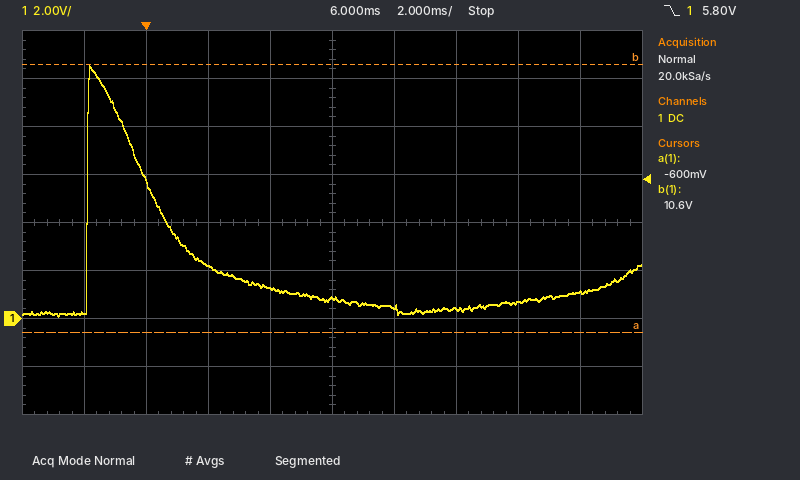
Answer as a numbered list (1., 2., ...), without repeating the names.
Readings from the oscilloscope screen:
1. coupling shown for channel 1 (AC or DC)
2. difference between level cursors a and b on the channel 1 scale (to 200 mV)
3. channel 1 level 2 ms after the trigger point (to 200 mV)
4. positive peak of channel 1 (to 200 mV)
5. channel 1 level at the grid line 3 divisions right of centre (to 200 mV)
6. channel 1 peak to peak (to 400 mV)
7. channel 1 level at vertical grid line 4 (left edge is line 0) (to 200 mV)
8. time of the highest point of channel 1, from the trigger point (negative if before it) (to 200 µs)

1. DC
2. 11.2 V
3. 2.2 V
4. 10.6 V
5. 600 mV
6. 10.4 V
7. 1.2 V
8. -1.8 ms
